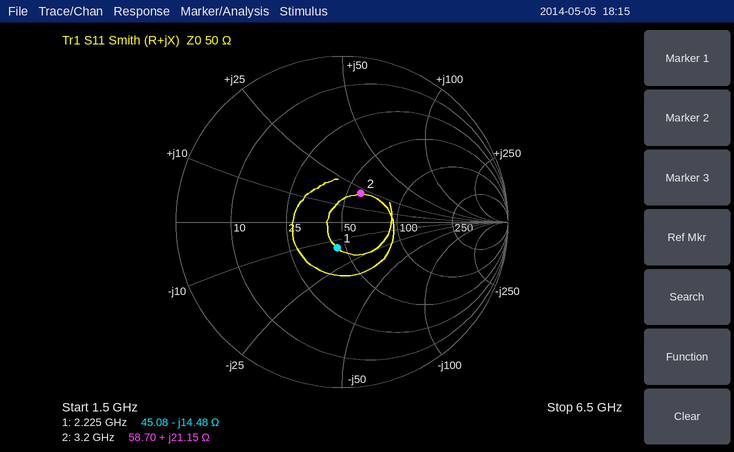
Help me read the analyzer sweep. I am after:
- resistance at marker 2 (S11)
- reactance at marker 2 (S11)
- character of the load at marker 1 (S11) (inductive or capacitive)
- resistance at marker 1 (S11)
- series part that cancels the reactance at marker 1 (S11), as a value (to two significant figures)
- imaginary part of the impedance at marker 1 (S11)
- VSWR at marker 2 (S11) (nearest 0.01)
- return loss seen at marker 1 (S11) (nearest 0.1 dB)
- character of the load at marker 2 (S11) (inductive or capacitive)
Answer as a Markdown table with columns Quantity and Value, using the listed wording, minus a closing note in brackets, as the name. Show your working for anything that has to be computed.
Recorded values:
| Quantity | Value |
|---|---|
| resistance at marker 2 | 58.70 Ω |
| reactance at marker 2 | +21.15 Ω |
| character of the load at marker 1 (S11) | capacitive |
| resistance at marker 1 | 45.08 Ω |
| series part that cancels the reactance at marker 1 (S11), as a value | L = 14.48 Ω/(2π × 2.225 GHz) ≈ 1.0 nH |
| imaginary part of the impedance at marker 1 | -14.48 Ω |
| VSWR at marker 2 (S11) | 1.52 |
| return loss seen at marker 1 (S11) | 16.0 dB |
| character of the load at marker 2 (S11) | inductive |
